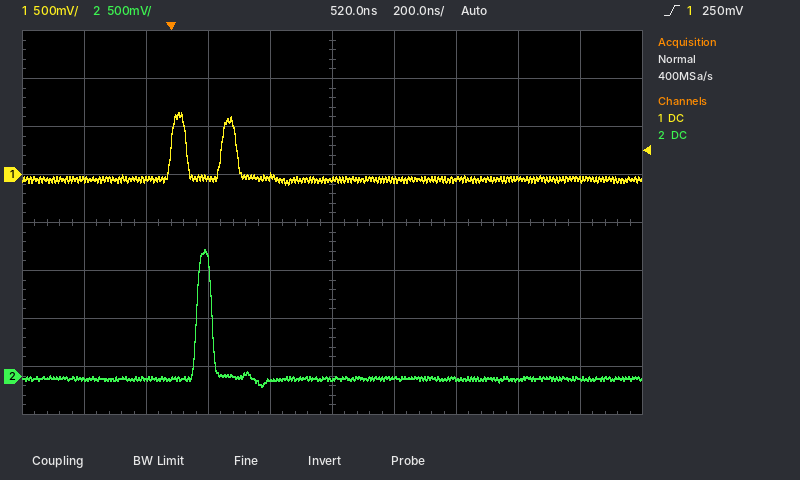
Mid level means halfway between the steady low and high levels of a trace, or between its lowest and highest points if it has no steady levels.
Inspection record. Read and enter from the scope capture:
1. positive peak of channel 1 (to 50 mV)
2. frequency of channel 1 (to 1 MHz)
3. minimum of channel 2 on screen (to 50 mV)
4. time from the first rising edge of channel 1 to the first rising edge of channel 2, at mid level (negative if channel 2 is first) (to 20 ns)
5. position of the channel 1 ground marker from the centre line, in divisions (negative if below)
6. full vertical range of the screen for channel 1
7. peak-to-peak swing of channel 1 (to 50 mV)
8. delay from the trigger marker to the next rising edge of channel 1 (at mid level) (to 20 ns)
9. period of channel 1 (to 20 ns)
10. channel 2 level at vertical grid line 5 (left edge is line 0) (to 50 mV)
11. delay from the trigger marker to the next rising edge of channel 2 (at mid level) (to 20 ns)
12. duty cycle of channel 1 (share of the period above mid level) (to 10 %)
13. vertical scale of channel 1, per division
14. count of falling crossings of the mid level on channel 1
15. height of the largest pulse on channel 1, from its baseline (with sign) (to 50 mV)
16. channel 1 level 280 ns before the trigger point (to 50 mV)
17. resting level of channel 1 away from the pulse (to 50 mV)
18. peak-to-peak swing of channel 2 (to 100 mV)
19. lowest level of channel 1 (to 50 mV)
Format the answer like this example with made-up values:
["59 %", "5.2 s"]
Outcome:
["650 mV", "6 MHz", "-100 mV", "+80 ns", "+1.0 div", "4 V", "750 mV", "160 ns", "160 ns", "-50 mV", "80 ns", "30 %", "500 mV", "2", "+700 mV", "-50 mV", "-50 mV", "1.40 V", "-100 mV"]
